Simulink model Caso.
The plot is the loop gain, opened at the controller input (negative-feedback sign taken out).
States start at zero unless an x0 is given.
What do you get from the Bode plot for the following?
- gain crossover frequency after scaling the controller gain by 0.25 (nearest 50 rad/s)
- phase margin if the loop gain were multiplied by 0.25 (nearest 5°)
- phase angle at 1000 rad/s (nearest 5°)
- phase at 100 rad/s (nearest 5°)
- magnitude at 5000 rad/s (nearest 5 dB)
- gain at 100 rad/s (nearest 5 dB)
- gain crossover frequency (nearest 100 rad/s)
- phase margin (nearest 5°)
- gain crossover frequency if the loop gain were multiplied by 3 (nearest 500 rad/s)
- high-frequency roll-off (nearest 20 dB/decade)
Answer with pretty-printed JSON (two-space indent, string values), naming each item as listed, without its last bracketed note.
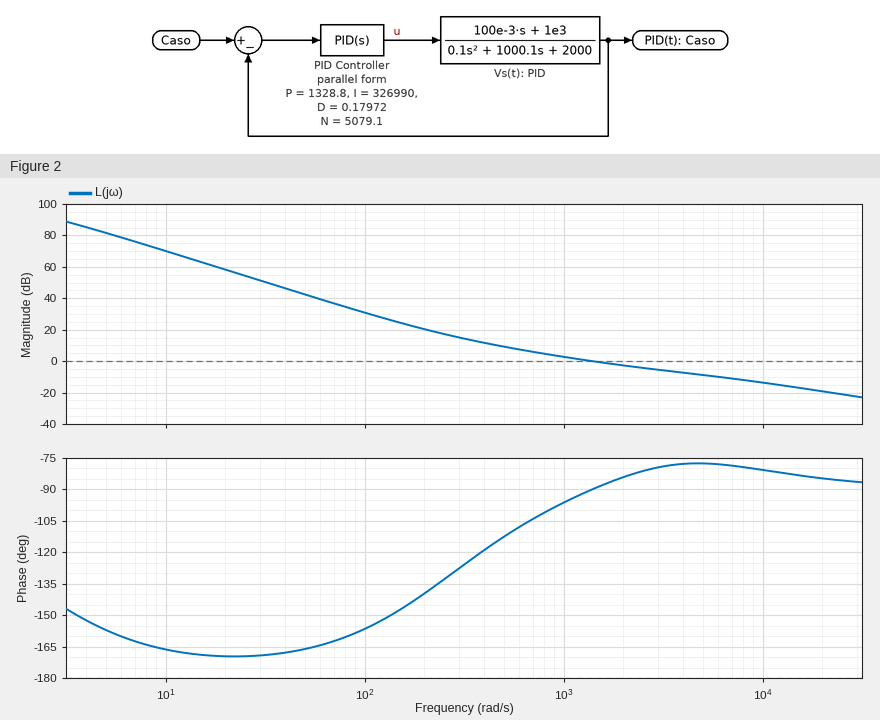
{
  "gain crossover frequency after scaling the controller gain by 0.25": "400 rad/s",
  "phase margin if the loop gain were multiplied by 0.25": "60°",
  "phase angle at 1000 rad/s": "-95°",
  "phase at 100 rad/s": "-155°",
  "magnitude at 5000 rad/s": "-10 dB",
  "gain at 100 rad/s": "30 dB",
  "gain crossover frequency": "1400 rad/s",
  "phase margin": "90°",
  "gain crossover frequency if the loop gain were multiplied by 3": "5500 rad/s",
  "high-frequency roll-off": "-20 dB/decade"
}
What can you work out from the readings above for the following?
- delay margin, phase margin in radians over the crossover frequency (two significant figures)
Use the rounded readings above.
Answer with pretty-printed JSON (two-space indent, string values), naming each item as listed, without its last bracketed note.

{
  "delay margin, phase margin in radians over the crossover frequency": "0.0011 s"
}
